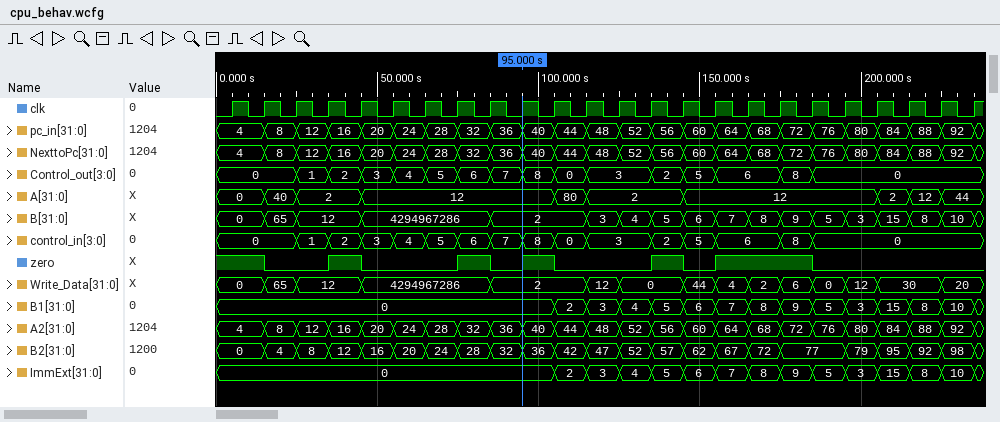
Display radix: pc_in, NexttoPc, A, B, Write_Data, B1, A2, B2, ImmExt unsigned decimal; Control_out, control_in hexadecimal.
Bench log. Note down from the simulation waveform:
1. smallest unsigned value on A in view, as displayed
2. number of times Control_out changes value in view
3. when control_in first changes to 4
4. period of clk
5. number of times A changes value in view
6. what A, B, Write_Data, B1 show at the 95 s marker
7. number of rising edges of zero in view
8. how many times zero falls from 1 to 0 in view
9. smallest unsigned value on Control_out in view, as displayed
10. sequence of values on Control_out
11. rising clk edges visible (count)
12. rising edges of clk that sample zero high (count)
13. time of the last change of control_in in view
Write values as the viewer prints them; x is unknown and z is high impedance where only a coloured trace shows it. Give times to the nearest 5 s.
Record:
0
15
55 s
10 s
9
A=12, B=2, Write_Data=2, B1=0
5
6
0
0, 1, 2, 3, 4, 5, 6, 7, 8, 0, 3, 2, 5, 6, 8, 0
24
9
185 s
